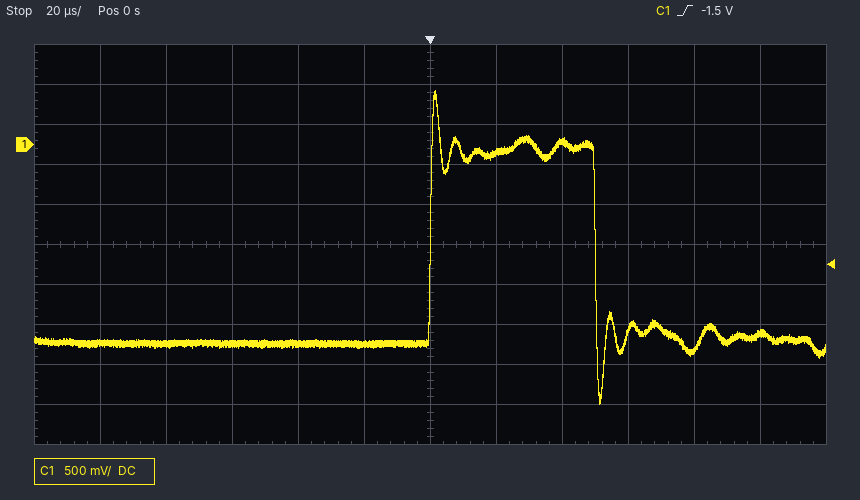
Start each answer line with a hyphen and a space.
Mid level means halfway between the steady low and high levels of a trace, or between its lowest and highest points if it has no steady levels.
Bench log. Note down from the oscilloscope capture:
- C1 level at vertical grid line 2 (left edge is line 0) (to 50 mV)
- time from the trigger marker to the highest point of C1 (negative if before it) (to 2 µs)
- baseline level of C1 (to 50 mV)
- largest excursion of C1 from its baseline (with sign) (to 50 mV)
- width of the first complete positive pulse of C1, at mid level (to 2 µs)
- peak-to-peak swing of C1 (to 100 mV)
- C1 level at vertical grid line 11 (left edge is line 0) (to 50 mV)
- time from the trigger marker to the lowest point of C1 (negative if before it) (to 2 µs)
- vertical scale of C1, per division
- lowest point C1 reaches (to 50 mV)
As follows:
- -2.50 V
- +2 µs
- -2.50 V
- +3.15 V
- 50 µs
- 3.90 V
- -2.35 V
- +52 µs
- 500 mV
- -3.25 V
